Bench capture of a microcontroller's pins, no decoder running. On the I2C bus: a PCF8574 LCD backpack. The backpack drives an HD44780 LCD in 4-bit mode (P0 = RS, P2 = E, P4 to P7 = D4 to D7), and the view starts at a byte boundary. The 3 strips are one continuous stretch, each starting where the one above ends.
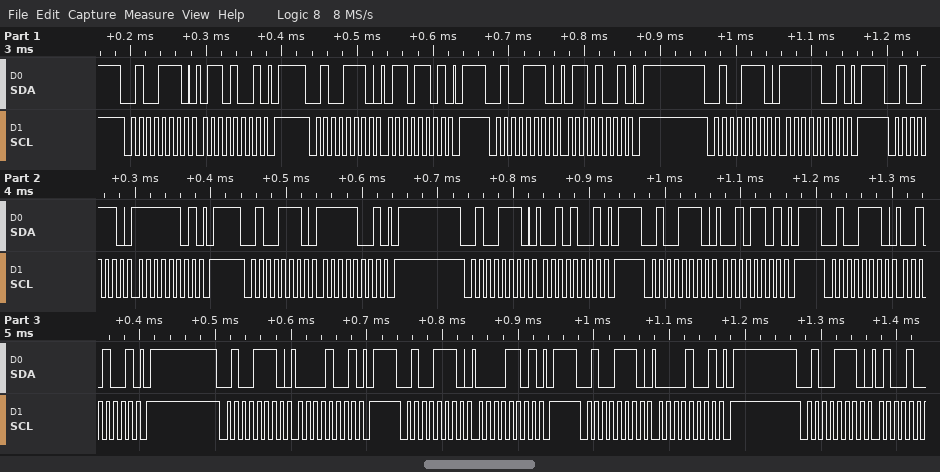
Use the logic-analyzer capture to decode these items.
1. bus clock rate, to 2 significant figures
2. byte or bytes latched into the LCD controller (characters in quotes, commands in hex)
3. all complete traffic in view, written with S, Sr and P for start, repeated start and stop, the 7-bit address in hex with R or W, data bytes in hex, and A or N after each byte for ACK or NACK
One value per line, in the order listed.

100 kHz
'o' ' '
S 27W A 69 A P S 27W A 6D A P S 27W A 69 A P S 27W A F9 A P S 27W A FD A P S 27W A F9 A P S 27W A 29 A P S 27W A 2D A P S 27W A 29 A P S 27W A 09 A P S 27W A 0D A P S 27W A 09 A P S 27W A
